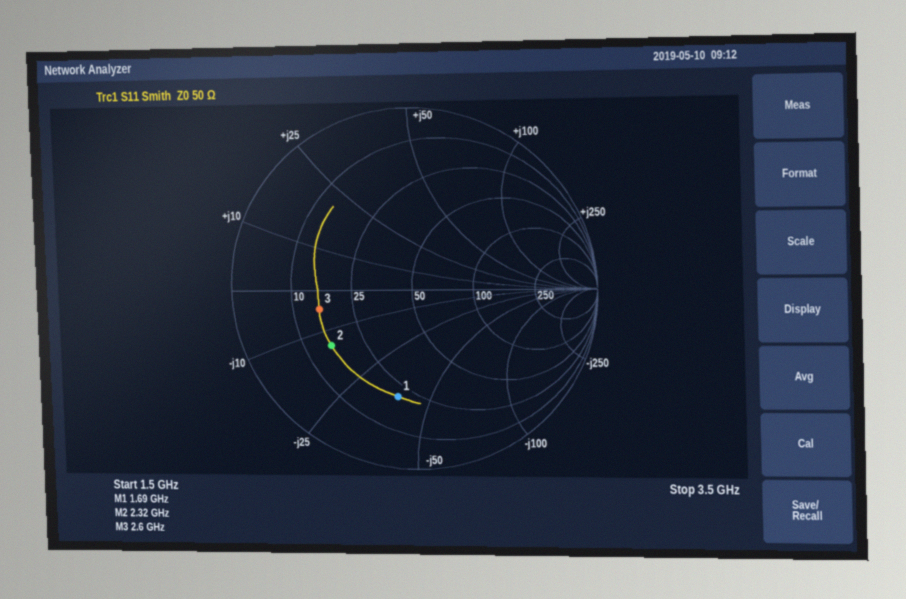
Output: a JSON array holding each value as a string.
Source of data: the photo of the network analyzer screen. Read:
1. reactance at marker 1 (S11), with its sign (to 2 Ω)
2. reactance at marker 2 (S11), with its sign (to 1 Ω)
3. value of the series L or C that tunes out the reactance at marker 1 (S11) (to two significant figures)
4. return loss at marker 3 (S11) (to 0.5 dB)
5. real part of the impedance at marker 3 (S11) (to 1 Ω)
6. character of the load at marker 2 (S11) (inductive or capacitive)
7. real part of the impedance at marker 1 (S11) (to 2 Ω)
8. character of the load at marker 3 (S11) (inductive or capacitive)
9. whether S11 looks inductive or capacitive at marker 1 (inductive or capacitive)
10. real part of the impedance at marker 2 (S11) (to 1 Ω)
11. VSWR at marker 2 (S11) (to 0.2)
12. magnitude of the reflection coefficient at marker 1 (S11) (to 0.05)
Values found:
["-38 Ω", "-14 Ω", "3.6 nH", "5.5 dB", "16 Ω", "capacitive", "20 Ω", "capacitive", "capacitive", "16 Ω", "3.4", "0.60"]
